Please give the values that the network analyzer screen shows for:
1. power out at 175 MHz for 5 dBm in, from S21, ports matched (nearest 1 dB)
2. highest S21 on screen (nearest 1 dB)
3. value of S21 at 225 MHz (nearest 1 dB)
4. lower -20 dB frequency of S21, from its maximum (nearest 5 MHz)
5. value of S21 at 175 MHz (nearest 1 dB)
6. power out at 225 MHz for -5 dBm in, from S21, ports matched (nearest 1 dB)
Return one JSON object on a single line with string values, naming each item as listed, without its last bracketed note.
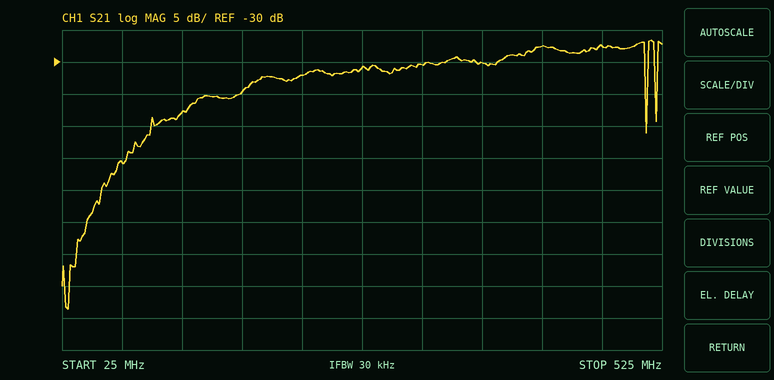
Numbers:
{"power out at 175 MHz for 5 dBm in, from S21, ports matched": "-30 dBm", "highest S21 on screen": "-27 dB", "value of S21 at 225 MHz": "-32 dB", "lower -20 dB frequency of S21, from its maximum": "70 MHz", "value of S21 at 175 MHz": "-35 dB", "power out at 225 MHz for -5 dBm in, from S21, ports matched": "-37 dBm"}
